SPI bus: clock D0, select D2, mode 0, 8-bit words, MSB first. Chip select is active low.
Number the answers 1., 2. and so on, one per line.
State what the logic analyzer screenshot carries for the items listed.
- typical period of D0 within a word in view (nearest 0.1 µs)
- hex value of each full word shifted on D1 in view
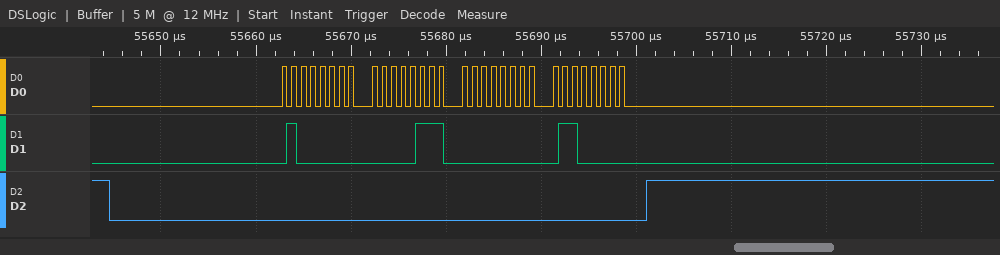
1. 1 µs
2. 40, 07, 00, 60
